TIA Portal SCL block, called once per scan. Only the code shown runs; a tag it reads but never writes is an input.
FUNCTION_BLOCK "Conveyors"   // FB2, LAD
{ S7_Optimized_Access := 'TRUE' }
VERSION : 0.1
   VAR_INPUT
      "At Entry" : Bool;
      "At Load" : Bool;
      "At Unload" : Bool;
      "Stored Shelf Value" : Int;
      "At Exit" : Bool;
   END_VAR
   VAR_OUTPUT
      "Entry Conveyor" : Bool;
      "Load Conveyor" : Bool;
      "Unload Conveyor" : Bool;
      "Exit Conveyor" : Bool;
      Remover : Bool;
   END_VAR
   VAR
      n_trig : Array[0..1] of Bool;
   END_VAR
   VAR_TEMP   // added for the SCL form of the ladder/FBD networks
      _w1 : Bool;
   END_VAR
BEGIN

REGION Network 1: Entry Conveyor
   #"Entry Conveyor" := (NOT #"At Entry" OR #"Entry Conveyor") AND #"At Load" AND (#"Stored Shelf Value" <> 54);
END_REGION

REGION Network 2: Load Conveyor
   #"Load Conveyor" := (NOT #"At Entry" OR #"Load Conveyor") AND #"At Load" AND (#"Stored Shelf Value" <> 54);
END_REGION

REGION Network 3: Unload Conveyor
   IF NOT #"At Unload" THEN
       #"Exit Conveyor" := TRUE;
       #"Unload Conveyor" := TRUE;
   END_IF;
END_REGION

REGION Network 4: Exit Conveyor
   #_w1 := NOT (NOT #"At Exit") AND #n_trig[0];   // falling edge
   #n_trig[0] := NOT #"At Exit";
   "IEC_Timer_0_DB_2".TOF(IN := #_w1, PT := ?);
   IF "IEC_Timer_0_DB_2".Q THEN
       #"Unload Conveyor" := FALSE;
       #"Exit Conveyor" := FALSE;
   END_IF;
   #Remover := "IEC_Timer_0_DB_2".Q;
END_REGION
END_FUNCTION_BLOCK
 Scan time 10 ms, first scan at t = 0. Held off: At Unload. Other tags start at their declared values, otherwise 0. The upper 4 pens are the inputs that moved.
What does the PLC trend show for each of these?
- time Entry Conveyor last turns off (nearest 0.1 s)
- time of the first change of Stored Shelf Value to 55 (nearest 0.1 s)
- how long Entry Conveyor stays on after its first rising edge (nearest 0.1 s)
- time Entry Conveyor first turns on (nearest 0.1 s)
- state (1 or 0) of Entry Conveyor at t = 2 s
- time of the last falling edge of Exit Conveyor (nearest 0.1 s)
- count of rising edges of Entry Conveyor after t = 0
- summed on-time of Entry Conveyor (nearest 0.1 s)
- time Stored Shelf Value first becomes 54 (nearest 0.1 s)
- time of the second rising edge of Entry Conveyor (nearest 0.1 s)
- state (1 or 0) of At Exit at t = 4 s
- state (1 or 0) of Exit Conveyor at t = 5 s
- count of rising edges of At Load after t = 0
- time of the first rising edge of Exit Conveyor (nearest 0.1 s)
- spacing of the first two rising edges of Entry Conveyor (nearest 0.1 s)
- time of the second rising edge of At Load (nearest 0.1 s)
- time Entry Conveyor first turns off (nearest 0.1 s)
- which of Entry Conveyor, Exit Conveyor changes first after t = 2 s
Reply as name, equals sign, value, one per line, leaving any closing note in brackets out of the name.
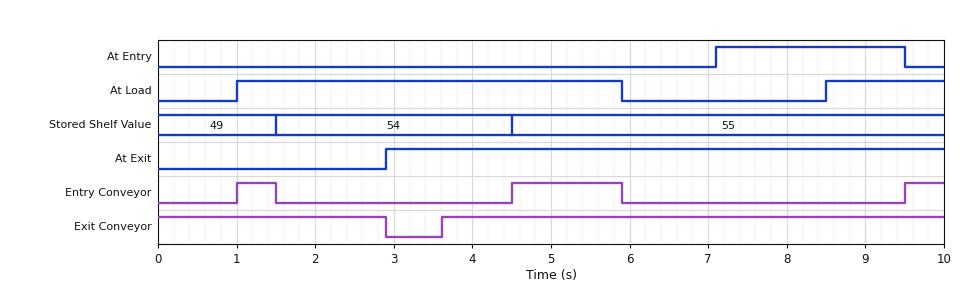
time Entry Conveyor last turns off = 5.9 s
time of the first change of Stored Shelf Value to 55 = 4.5 s
how long Entry Conveyor stays on after its first rising edge = 0.5 s
time Entry Conveyor first turns on = 1.0 s
state (1 or 0) of Entry Conveyor at t = 2 s = 0
time of the last falling edge of Exit Conveyor = 2.9 s
count of rising edges of Entry Conveyor after t = 0 = 3
summed on-time of Entry Conveyor = 2.4 s
time Stored Shelf Value first becomes 54 = 1.5 s
time of the second rising edge of Entry Conveyor = 4.5 s
state (1 or 0) of At Exit at t = 4 s = 1
state (1 or 0) of Exit Conveyor at t = 5 s = 1
count of rising edges of At Load after t = 0 = 2
time of the first rising edge of Exit Conveyor = 3.6 s
spacing of the first two rising edges of Entry Conveyor = 3.5 s
time of the second rising edge of At Load = 8.5 s
time Entry Conveyor first turns off = 1.5 s
which of Entry Conveyor, Exit Conveyor changes first after t = 2 s = Exit Conveyor
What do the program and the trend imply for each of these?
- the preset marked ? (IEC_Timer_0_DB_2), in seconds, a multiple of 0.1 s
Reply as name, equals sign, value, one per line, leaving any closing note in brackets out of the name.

the preset marked ? (IEC_Timer_0_DB_2), in seconds, a multiple of 0.1 s = 0.7 s
